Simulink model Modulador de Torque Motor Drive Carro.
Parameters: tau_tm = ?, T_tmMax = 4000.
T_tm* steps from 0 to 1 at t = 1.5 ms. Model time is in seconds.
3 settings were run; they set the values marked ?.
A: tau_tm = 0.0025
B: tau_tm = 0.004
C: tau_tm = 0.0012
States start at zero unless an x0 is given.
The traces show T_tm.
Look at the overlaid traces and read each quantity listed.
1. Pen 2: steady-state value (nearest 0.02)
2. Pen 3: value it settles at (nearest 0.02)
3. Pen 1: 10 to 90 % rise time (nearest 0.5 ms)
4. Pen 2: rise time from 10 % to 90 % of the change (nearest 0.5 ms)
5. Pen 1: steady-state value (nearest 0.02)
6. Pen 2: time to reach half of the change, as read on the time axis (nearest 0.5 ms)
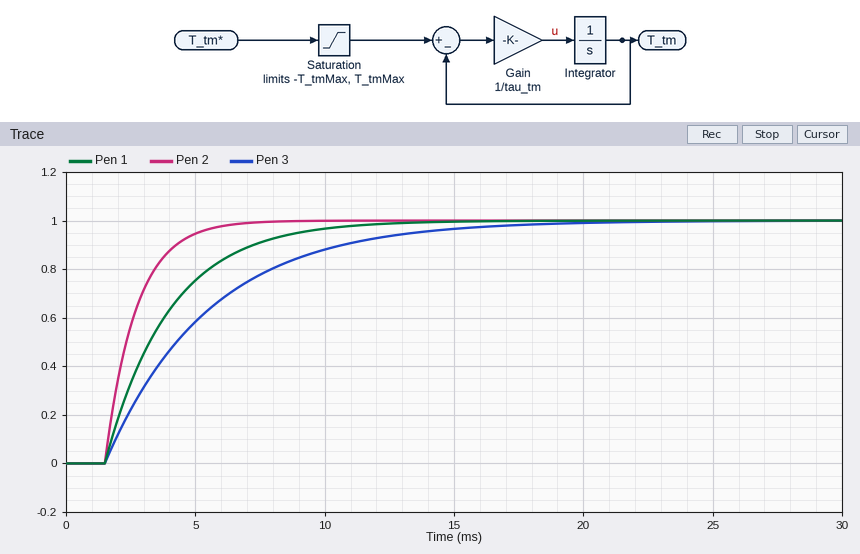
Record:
1.00
1.00
5.5 ms
2.5 ms
1.00
2.5 ms
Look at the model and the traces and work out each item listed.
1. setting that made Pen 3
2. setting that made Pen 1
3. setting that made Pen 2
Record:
B
A
C
